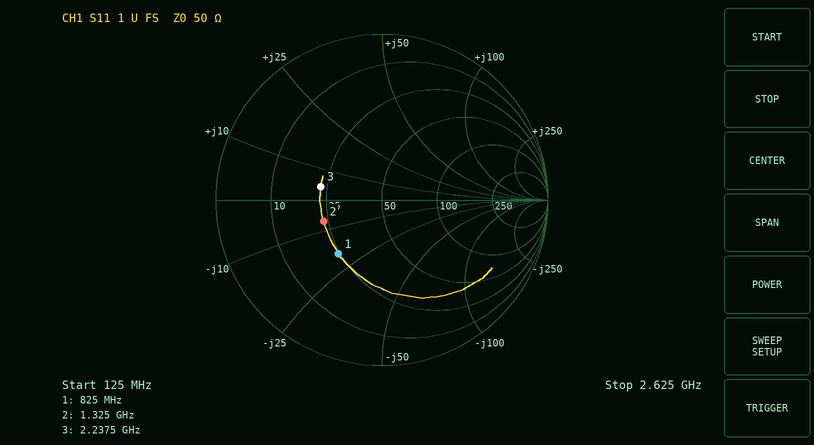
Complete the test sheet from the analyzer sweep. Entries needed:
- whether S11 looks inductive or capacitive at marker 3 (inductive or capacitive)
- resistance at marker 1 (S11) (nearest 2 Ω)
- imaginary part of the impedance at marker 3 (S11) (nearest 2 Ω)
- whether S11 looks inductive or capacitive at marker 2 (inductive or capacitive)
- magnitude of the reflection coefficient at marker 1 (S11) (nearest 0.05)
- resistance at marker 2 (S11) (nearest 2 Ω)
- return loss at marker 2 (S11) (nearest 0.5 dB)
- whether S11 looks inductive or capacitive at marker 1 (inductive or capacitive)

inductive
24 Ω
+4 Ω
capacitive
0.40
24 Ω
8.5 dB
capacitive
